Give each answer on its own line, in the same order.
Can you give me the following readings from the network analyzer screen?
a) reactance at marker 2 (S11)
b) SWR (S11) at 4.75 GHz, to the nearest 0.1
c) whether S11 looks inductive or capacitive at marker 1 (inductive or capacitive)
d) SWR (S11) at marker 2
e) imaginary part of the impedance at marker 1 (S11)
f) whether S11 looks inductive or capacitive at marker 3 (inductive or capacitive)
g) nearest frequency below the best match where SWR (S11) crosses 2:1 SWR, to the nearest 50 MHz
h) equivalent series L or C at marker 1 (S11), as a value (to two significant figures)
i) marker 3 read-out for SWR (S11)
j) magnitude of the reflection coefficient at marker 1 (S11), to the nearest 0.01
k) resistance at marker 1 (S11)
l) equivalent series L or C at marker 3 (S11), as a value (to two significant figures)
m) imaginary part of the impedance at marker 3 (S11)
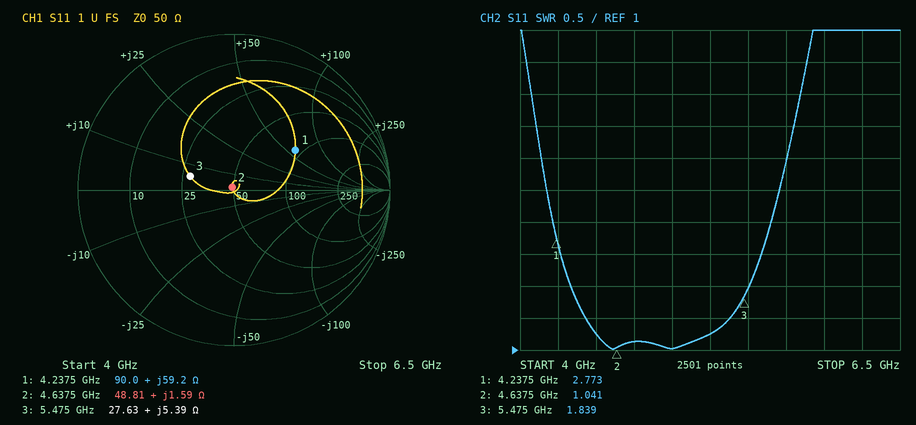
+1.59 Ω
1.1
inductive
1.041
+59.2 Ω
inductive
4.35 GHz
2.2 nH
1.839
0.47
90.0 Ω
160 pH
+5.39 Ω
